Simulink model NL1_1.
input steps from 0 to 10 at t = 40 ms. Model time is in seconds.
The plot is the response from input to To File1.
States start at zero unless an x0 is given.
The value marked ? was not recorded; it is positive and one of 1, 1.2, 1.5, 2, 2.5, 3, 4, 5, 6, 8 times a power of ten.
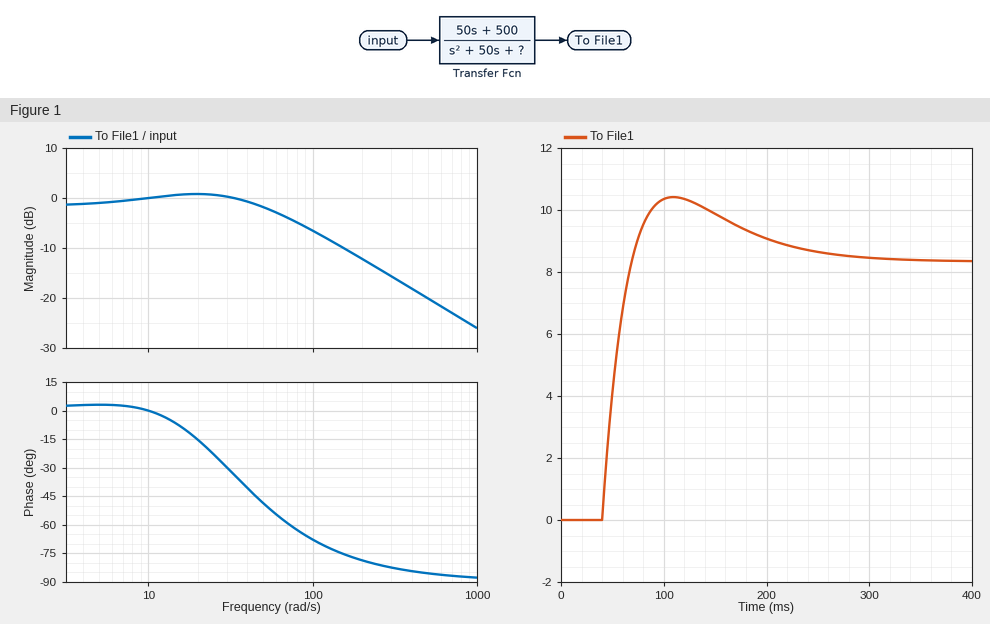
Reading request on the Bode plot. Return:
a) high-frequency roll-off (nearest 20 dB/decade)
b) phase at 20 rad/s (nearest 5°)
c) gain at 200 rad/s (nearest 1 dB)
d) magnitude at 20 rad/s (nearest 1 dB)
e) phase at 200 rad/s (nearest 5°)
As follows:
-20 dB/decade
-15°
-12 dB
1 dB
-80°
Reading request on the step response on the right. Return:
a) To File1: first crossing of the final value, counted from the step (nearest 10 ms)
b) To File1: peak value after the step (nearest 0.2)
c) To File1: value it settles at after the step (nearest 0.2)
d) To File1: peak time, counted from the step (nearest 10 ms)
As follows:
30 ms
10.4
8.4
70 ms
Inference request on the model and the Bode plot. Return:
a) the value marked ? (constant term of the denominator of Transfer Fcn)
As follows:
600
